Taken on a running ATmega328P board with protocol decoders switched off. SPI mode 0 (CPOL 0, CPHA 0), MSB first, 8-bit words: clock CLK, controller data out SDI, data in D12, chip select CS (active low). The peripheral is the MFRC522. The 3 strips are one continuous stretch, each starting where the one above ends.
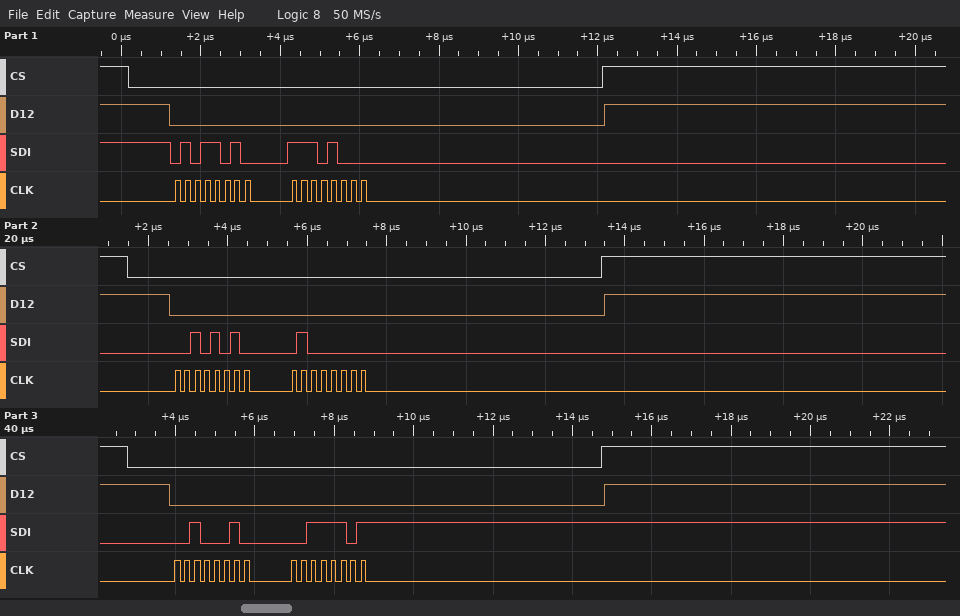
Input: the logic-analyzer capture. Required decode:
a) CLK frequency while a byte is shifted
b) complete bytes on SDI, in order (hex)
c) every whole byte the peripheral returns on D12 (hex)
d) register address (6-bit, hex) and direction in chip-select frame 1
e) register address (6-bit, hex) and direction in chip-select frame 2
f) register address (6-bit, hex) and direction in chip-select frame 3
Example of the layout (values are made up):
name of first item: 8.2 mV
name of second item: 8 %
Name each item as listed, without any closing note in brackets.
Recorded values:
CLK frequency while a byte is shifted: 4 MHz
complete bytes on SDI, in order: 5A E8 2A 40 22 3D
every whole byte the peripheral returns on D12: 00 00 00 00 00 00
register address (6-bit, hex) and direction in chip-select frame 1: 0x2D write
register address (6-bit, hex) and direction in chip-select frame 2: 0x15 write
register address (6-bit, hex) and direction in chip-select frame 3: 0x11 write
